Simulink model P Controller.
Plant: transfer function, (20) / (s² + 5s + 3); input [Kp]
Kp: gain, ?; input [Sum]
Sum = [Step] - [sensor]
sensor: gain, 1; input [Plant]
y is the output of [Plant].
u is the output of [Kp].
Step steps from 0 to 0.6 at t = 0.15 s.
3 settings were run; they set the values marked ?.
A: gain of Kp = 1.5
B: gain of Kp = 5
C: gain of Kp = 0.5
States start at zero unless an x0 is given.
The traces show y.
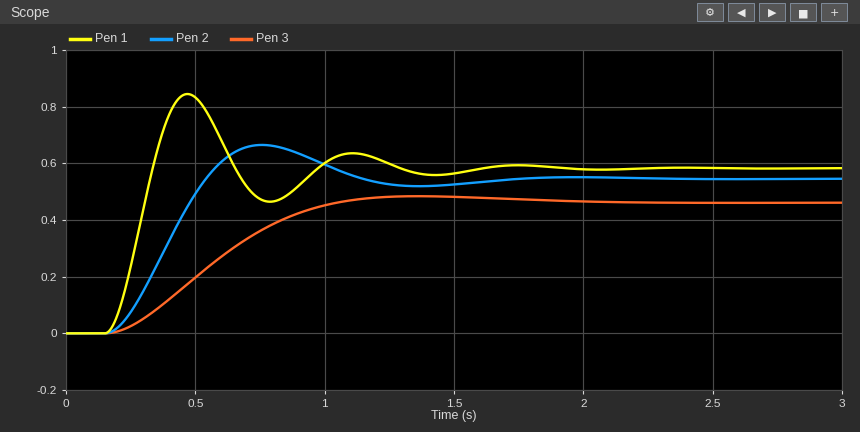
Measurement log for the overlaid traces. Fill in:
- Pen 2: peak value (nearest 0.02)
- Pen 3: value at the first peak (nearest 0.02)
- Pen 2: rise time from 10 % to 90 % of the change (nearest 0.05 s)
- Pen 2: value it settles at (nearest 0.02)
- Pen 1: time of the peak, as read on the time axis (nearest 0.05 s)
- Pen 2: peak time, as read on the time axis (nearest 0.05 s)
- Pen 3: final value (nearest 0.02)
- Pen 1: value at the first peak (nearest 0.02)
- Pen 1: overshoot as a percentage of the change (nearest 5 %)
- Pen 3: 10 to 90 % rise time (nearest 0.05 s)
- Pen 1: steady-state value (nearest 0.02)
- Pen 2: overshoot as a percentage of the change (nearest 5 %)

0.66
0.48
0.25 s
0.54
0.45 s
0.75 s
0.46
0.84
45 %
0.60 s
0.58
20 %
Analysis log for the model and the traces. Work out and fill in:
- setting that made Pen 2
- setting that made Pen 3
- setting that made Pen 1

A
C
B
